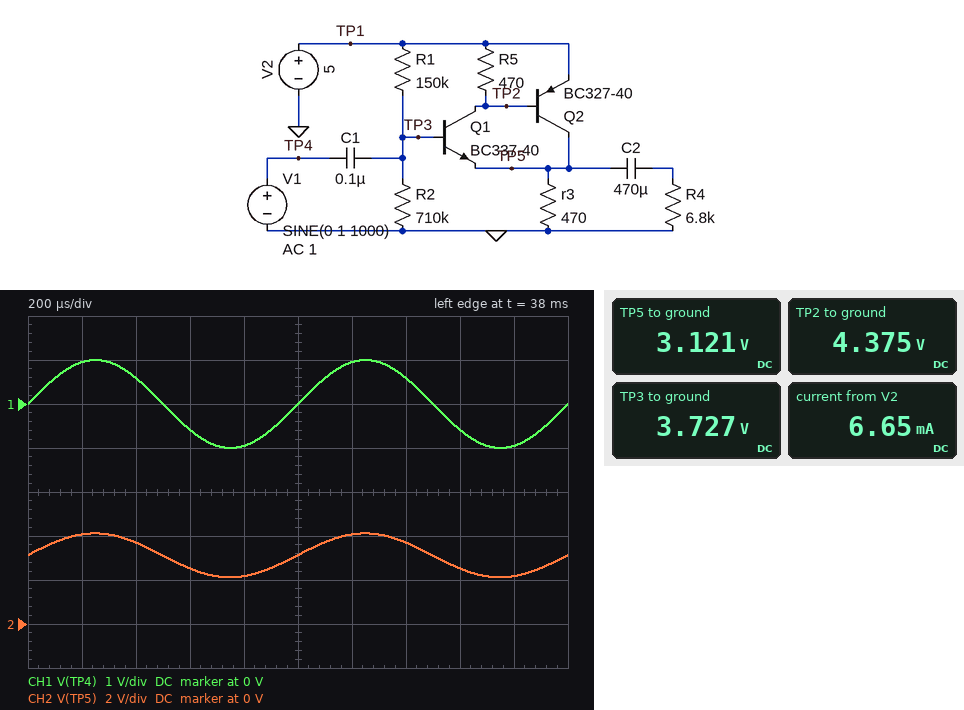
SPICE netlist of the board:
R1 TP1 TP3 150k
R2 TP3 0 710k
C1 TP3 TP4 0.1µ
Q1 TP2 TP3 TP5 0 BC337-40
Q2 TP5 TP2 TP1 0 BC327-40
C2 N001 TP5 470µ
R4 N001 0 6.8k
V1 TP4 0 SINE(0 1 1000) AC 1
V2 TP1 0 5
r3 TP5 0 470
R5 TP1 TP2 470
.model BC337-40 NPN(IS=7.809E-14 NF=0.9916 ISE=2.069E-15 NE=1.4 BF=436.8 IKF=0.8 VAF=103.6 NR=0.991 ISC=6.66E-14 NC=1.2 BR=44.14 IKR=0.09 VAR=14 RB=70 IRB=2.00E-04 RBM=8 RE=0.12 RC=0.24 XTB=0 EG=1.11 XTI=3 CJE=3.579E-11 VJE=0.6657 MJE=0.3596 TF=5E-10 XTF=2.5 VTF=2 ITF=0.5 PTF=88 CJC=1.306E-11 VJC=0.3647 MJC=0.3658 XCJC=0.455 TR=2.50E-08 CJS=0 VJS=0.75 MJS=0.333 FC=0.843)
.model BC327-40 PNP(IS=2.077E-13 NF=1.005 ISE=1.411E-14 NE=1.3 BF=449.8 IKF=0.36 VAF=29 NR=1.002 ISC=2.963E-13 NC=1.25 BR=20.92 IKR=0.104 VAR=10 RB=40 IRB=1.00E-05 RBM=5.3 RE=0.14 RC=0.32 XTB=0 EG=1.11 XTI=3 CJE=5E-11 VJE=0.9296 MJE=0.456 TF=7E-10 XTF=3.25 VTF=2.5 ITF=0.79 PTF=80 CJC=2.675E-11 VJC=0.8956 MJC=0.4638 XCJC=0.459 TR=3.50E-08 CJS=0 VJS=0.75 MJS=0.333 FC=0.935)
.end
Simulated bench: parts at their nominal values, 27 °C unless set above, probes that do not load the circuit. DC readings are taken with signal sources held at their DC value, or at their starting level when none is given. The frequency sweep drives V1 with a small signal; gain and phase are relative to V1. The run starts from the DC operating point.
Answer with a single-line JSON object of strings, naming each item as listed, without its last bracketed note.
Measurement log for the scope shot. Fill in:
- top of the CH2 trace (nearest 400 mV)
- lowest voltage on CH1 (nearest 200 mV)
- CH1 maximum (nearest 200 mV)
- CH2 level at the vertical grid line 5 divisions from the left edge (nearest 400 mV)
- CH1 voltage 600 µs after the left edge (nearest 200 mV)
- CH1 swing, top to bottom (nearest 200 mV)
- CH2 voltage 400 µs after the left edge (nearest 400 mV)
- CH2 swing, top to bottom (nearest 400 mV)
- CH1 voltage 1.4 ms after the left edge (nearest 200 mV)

{"top of the CH2 trace": "4.0 V", "lowest voltage on CH1": "-1.0 V", "CH1 maximum": "1.0 V", "CH2 level at the vertical grid line 5 divisions from the left edge": "3.2 V", "CH1 voltage 600 µs after the left edge": "-600 mV", "CH1 swing, top to bottom": "2.0 V", "CH2 voltage 400 µs after the left edge": "3.6 V", "CH2 swing, top to bottom": "2.0 V", "CH1 voltage 1.4 ms after the left edge": "600 mV"}
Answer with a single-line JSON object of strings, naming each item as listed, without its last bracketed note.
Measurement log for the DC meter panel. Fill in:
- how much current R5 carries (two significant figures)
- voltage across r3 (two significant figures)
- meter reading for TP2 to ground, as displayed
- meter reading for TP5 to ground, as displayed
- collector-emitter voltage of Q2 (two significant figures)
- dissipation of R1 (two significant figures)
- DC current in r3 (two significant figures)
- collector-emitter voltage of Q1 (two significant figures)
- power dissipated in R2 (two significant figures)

{"how much current R5 carries": "1.3 mA", "voltage across r3": "3.1 V", "meter reading for TP2 to ground, as displayed": "4.375 V", "meter reading for TP5 to ground, as displayed": "3.121 V", "collector-emitter voltage of Q2": "-1.9 V", "dissipation of R1": "11 µW", "DC current in r3": "6.6 mA", "collector-emitter voltage of Q1": "1.3 V", "power dissipated in R2": "20 µW"}
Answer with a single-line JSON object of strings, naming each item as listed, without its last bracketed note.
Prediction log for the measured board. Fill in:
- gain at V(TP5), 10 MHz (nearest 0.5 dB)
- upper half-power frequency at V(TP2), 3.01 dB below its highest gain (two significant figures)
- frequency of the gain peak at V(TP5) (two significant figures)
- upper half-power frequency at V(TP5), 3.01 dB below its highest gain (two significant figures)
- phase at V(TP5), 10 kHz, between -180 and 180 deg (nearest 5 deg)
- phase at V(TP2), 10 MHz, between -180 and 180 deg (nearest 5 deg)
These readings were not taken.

{"gain at V(TP5), 10 MHz": "0 dB", "upper half-power frequency at V(TP2), 3.01 dB below its highest gain": "62 MHz", "frequency of the gain peak at V(TP5)": "61 MHz", "upper half-power frequency at V(TP5), 3.01 dB below its highest gain": "62 MHz", "phase at V(TP5), 10 kHz, between -180 and 180 deg": "0 deg", "phase at V(TP2), 10 MHz, between -180 and 180 deg": "-145 deg"}
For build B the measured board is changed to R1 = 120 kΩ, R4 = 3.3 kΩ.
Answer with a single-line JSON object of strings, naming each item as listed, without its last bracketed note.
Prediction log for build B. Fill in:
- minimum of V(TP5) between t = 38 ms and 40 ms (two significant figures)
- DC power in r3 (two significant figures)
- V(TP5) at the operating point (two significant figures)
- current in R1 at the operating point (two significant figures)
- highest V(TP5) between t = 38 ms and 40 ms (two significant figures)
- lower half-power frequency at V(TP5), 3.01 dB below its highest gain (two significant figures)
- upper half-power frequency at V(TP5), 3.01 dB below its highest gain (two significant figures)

{"minimum of V(TP5) between t = 38 ms and 40 ms": "2.3 V", "DC power in r3": "24 mW", "V(TP5) at the operating point": "3.3 V", "current in R1 at the operating point": "8.8 µA", "highest V(TP5) between t = 38 ms and 40 ms": "4.3 V", "lower half-power frequency at V(TP5), 3.01 dB below its highest gain": "59 MHz", "upper half-power frequency at V(TP5), 3.01 dB below its highest gain": "61 MHz"}
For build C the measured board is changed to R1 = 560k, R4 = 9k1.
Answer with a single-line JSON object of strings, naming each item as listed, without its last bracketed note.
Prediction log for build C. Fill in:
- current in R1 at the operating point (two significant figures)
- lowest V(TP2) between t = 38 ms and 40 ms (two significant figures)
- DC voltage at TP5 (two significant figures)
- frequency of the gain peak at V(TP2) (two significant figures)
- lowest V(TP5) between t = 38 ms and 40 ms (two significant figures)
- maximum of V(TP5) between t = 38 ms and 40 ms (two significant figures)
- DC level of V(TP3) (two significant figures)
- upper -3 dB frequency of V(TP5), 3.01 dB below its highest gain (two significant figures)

{"current in R1 at the operating point": "5.6 µA", "lowest V(TP2) between t = 38 ms and 40 ms": "4.4 V", "DC voltage at TP5": "1.3 V", "frequency of the gain peak at V(TP2)": "54 MHz", "lowest V(TP5) between t = 38 ms and 40 ms": "340 mV", "maximum of V(TP5) between t = 38 ms and 40 ms": "2.3 V", "DC level of V(TP3)": "1.9 V", "upper -3 dB frequency of V(TP5), 3.01 dB below its highest gain": "56 MHz"}
